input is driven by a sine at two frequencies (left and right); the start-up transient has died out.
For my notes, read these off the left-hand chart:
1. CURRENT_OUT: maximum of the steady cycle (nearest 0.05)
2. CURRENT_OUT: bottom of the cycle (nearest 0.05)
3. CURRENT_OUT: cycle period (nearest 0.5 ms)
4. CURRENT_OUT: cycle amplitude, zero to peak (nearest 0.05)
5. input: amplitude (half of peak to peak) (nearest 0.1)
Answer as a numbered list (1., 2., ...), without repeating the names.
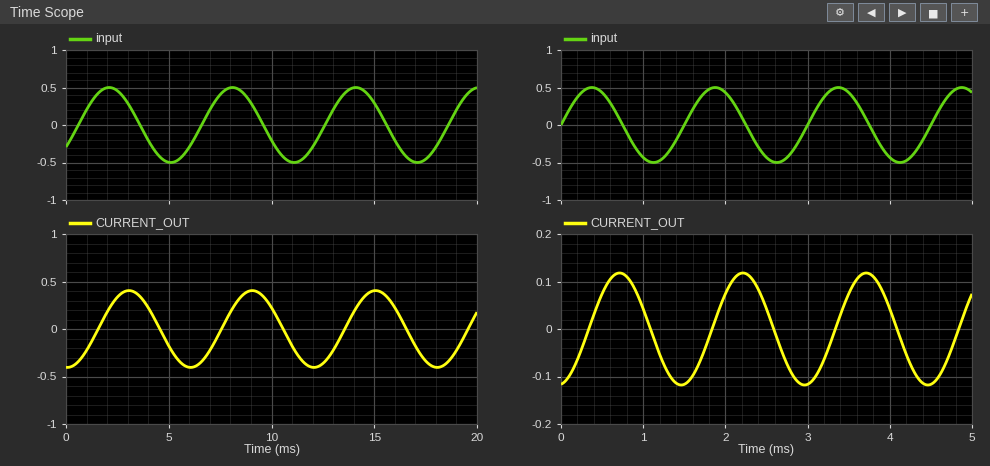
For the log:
1. 0.40
2. -0.40
3. 6.0 ms
4. 0.40
5. 0.5
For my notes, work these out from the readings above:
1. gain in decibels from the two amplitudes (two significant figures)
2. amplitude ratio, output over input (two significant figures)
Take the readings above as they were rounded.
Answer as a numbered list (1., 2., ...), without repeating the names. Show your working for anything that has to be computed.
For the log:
1. 20 log10(0.4 / 0.5) = -1.9 dB
2. 0.4 / 0.5 = 0.80
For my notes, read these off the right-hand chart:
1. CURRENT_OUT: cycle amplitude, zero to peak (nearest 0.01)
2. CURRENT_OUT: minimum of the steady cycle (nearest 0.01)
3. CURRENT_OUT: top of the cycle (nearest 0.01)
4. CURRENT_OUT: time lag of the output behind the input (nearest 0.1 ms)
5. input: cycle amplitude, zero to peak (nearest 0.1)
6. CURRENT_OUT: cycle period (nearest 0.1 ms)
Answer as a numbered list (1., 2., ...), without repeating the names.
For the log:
1. 0.12
2. -0.12
3. 0.12
4. 0.3 ms
5. 0.5
6. 1.5 ms
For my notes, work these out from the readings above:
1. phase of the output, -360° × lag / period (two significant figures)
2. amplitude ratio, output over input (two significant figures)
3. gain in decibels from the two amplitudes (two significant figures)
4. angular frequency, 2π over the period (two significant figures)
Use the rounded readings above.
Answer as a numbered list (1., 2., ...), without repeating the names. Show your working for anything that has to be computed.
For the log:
1. -360 × 0.3 / 1.5 = -72°
2. 0.12 / 0.5 = 0.24
3. 20 log10(0.12 / 0.5) = -12 dB
4. 2π / 1.5 = 4.2 rad/ms
